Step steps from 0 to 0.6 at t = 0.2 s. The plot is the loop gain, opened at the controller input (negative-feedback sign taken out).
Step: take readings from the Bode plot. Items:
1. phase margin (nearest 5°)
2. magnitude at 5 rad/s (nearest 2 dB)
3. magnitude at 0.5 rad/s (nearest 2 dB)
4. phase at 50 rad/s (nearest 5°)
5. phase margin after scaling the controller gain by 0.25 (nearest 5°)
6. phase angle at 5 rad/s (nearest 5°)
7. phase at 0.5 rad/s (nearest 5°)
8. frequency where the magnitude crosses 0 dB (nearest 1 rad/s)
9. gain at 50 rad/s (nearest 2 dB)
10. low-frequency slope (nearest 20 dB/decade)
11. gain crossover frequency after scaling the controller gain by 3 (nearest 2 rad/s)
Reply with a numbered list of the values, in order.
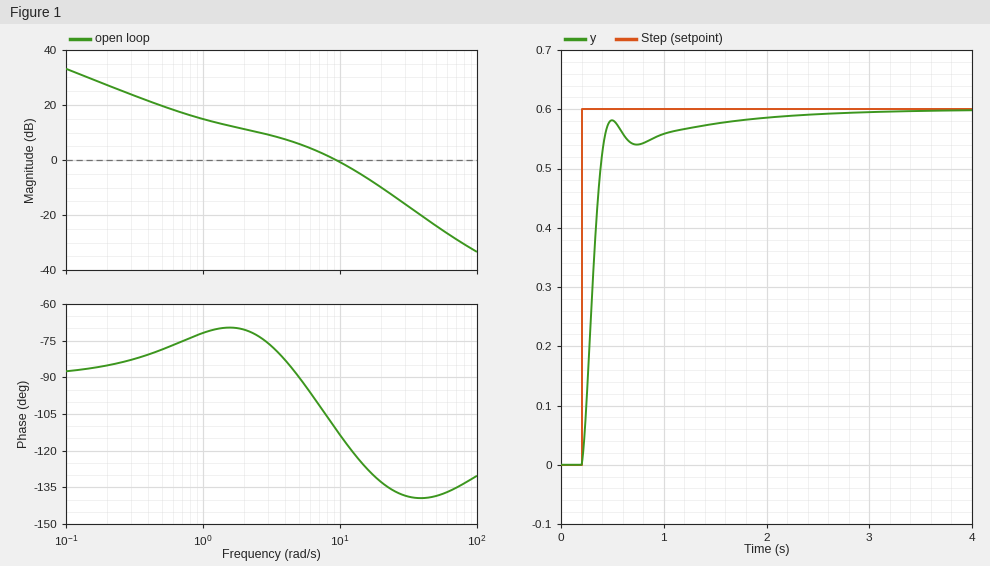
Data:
1. 70°
2. 6 dB
3. 20 dB
4. -140°
5. 110°
6. -90°
7. -80°
8. 9 rad/s
9. -24 dB
10. -20 dB/decade
11. 20 rad/s
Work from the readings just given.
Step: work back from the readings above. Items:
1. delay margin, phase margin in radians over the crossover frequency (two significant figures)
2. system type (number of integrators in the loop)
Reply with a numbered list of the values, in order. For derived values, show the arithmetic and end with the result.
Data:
1. 70 × π / 180 / 9 = 0.14 s
2. 1
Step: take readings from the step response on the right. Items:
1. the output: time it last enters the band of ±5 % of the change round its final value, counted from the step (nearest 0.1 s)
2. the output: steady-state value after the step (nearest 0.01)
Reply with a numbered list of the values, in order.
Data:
1. 1.1 s
2. 0.60
